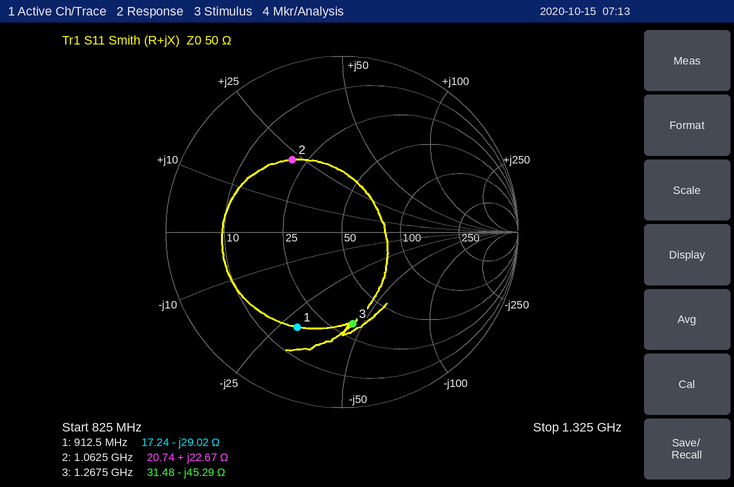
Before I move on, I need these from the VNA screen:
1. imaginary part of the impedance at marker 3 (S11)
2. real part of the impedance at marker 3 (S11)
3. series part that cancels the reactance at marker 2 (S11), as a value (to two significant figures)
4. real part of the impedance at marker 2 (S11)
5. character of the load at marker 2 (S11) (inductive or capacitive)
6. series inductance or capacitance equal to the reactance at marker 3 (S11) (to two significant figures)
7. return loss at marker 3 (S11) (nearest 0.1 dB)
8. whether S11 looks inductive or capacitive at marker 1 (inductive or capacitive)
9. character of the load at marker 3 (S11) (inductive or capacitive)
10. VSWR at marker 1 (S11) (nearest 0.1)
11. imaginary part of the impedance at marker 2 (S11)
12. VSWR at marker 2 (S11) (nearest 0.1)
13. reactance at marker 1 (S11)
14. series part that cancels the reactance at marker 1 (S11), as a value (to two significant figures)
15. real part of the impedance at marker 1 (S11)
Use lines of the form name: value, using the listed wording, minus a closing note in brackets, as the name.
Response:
imaginary part of the impedance at marker 3: -45.29 Ω
real part of the impedance at marker 3: 31.48 Ω
series part that cancels the reactance at marker 2 (S11), as a value: 6.6 pF
real part of the impedance at marker 2: 20.74 Ω
character of the load at marker 2 (S11): inductive
series inductance or capacitance equal to the reactance at marker 3 (S11): 2.8 pF
return loss at marker 3 (S11): 5.6 dB
whether S11 looks inductive or capacitive at marker 1: capacitive
character of the load at marker 3 (S11): capacitive
VSWR at marker 1 (S11): 4.0
imaginary part of the impedance at marker 2: +22.67 Ω
VSWR at marker 2 (S11): 3.0
reactance at marker 1: -29.02 Ω
series part that cancels the reactance at marker 1 (S11), as a value: 5.1 nH
real part of the impedance at marker 1: 17.24 Ω
